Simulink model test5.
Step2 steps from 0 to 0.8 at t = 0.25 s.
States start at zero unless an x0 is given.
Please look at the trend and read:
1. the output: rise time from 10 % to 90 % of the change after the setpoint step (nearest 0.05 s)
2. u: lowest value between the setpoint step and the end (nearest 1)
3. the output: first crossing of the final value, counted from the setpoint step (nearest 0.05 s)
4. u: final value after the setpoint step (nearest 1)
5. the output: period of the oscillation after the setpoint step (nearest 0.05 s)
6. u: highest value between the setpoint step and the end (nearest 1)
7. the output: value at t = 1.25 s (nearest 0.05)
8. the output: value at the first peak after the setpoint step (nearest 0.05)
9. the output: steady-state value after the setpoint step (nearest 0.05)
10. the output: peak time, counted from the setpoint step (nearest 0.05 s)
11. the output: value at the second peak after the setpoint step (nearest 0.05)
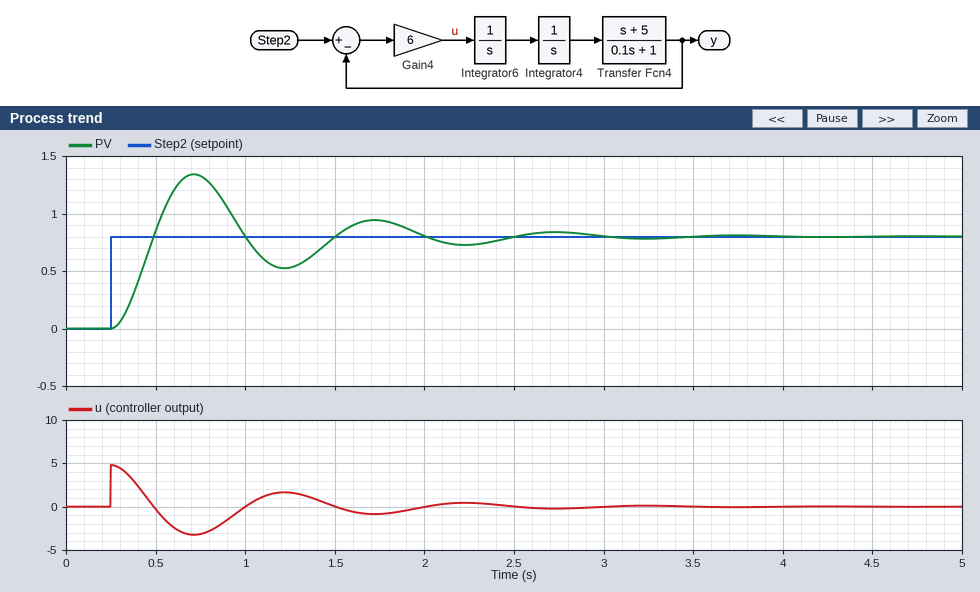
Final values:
0.15 s
-3
0.25 s
0
1.00 s
5
0.55
1.35
0.80
0.45 s
0.95
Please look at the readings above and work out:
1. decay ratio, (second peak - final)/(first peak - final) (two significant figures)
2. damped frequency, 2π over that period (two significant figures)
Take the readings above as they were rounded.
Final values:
0.27
6.3 rad/s
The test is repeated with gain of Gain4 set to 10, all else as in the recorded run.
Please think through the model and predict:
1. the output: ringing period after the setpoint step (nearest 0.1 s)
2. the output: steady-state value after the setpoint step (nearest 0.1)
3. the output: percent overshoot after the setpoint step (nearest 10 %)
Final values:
0.7 s
0.8
70 %
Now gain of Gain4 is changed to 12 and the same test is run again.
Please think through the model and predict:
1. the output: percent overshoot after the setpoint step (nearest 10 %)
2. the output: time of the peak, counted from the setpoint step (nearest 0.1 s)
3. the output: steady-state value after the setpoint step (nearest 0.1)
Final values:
70 %
0.3 s
0.8
